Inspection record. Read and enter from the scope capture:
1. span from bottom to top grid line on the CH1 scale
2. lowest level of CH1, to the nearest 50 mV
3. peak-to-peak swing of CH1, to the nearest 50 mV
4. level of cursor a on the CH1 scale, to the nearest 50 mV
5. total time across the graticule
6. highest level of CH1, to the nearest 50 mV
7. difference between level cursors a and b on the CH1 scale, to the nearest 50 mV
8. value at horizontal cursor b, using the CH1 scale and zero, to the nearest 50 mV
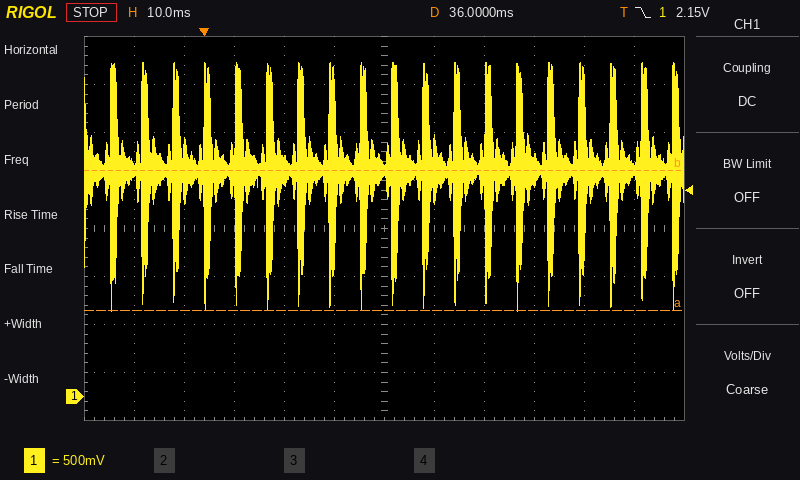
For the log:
4 V
900 mV
2.60 V
900 mV
120 ms
3.50 V
1.45 V
2.35 V
